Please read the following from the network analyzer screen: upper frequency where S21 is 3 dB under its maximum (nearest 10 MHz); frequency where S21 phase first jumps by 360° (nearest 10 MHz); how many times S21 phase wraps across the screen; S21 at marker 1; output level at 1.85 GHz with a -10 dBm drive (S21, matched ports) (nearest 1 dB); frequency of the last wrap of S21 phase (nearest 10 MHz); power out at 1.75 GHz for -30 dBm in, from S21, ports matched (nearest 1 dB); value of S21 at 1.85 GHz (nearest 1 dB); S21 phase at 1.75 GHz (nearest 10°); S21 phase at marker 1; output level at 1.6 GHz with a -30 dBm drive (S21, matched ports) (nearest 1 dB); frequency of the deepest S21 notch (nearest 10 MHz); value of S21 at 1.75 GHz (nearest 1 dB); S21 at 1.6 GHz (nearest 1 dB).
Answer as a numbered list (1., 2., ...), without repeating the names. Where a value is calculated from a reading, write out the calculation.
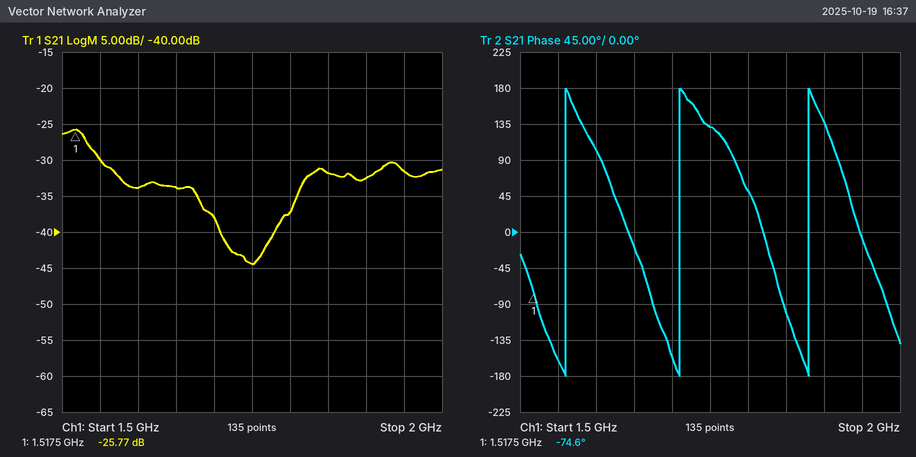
1. 1.54 GHz
2. 1.56 GHz
3. 3
4. -25.77 dB
5. -10 dBm + (-32 dB) = -42 dBm
6. 1.88 GHz
7. -30 dBm + (-44 dB) = -74 dBm
8. -32 dB
9. 130°
10. -74.6°
11. -30 dBm + (-34 dB) = -64 dBm
12. 1.75 GHz
13. -44 dB
14. -34 dB
